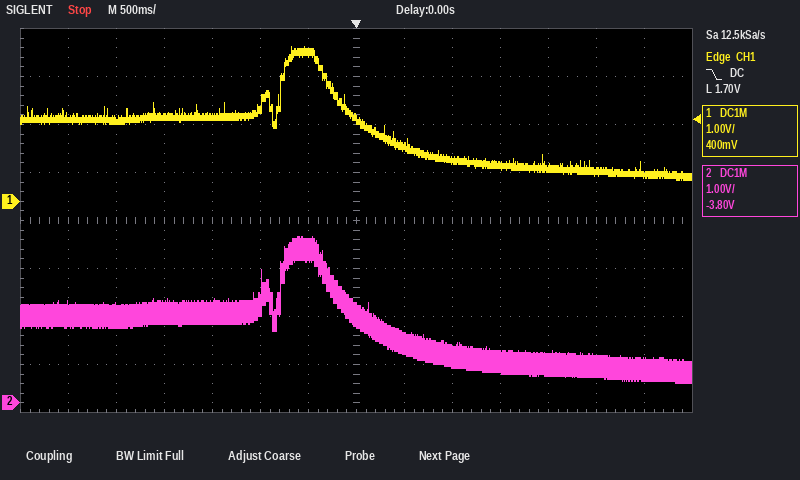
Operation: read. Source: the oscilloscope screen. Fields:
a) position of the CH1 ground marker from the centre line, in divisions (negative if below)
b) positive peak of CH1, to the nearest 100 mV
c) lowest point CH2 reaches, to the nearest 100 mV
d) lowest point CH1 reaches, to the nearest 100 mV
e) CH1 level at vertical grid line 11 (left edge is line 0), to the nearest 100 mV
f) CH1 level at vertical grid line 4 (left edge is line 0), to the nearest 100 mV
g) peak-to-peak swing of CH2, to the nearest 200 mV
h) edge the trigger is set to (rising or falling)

+0.4 div
3.2 V
400 mV
500 mV
700 mV
1.8 V
3.0 V
falling
